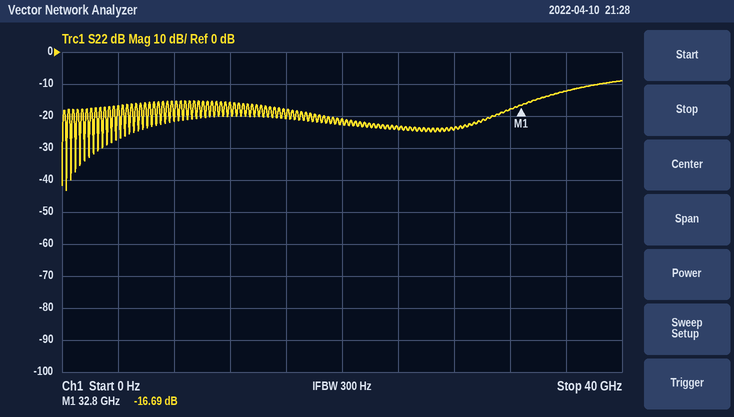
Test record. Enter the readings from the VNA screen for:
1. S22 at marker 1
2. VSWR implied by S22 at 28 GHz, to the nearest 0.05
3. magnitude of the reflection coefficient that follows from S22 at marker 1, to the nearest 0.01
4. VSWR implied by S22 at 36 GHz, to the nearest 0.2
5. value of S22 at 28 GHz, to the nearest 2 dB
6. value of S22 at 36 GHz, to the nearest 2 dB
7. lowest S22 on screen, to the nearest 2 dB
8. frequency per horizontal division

-16.69 dB
1.15
0.15
1.6
-24 dB
-12 dB
-44 dB
4 GHz
